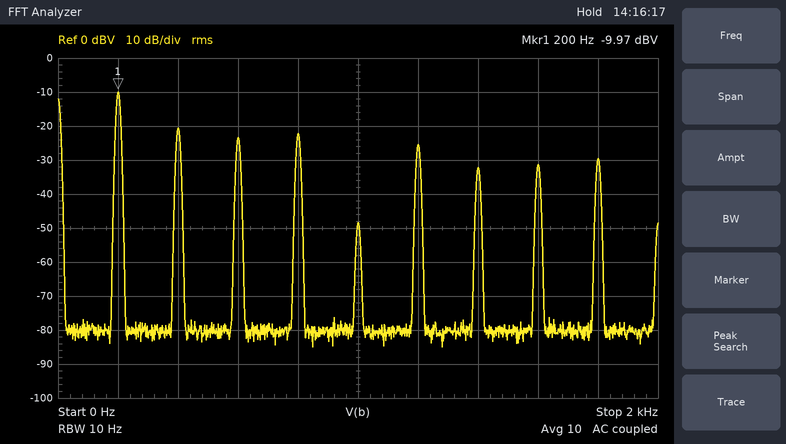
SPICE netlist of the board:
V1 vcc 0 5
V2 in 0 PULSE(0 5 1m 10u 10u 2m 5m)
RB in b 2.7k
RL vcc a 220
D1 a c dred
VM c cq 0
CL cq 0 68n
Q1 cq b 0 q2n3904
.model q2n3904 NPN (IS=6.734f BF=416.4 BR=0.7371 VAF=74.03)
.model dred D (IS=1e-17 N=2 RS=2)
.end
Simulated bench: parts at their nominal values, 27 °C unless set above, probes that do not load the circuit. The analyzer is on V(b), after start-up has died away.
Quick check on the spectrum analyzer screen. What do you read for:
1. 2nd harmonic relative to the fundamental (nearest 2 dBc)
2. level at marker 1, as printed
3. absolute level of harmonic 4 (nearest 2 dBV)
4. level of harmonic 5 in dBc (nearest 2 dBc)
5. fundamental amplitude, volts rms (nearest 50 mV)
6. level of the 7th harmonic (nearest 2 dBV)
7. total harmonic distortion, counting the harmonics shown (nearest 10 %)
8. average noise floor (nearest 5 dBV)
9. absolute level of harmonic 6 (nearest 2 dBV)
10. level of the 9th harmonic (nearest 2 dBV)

-10 dBc
-9.97 dBV
-22 dBV
-38 dBc
300 mV
-32 dBV
50 %
-80 dBV
-26 dBV
-30 dBV
